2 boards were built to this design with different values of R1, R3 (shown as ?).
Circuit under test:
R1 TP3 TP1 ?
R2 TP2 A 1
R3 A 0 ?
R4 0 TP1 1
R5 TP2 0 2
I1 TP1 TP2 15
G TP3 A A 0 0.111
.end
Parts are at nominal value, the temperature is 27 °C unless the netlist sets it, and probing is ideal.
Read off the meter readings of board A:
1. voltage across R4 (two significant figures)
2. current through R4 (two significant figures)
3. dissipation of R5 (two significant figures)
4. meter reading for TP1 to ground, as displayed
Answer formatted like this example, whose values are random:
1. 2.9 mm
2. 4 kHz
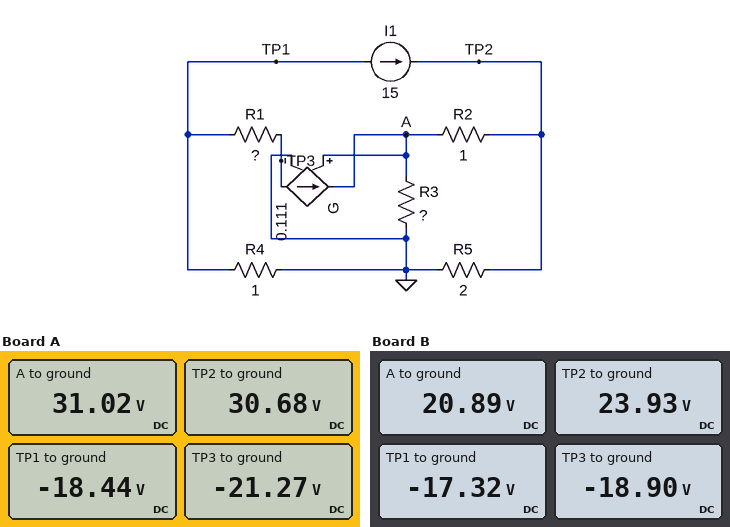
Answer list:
1. 18 V
2. 18 A
3. 470 W
4. -18.44 V
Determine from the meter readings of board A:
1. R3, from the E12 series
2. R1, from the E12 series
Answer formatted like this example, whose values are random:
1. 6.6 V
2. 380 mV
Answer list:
1. 10 Ω
2. 0.82 Ω
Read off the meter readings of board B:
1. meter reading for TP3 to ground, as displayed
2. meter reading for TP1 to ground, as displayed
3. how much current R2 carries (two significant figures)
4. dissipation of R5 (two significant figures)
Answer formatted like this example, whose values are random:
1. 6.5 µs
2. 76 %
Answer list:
1. -18.90 V
2. -17.32 V
3. 3.0 A
4. 290 W
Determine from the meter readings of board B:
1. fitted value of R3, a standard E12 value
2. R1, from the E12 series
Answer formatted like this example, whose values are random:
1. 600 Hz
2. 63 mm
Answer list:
1. 3.9 Ω
2. 0.68 Ω
